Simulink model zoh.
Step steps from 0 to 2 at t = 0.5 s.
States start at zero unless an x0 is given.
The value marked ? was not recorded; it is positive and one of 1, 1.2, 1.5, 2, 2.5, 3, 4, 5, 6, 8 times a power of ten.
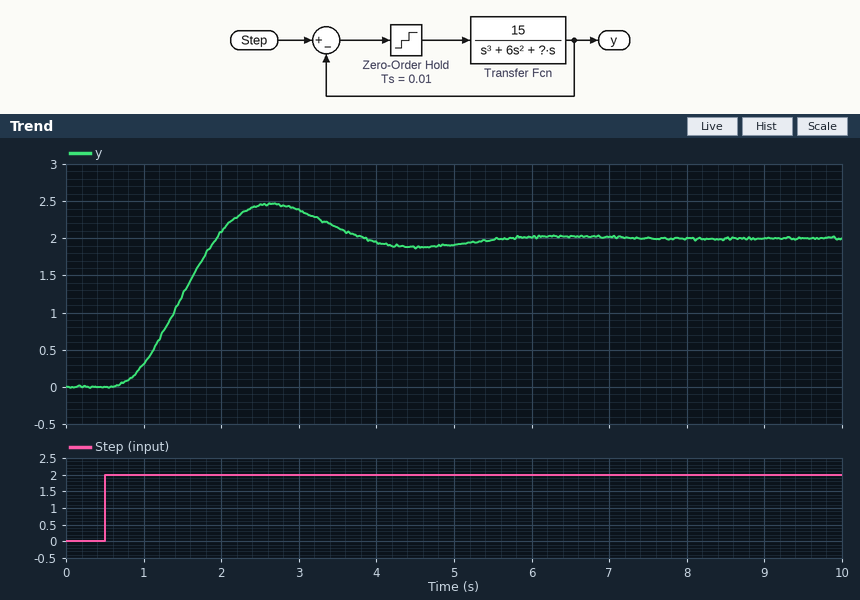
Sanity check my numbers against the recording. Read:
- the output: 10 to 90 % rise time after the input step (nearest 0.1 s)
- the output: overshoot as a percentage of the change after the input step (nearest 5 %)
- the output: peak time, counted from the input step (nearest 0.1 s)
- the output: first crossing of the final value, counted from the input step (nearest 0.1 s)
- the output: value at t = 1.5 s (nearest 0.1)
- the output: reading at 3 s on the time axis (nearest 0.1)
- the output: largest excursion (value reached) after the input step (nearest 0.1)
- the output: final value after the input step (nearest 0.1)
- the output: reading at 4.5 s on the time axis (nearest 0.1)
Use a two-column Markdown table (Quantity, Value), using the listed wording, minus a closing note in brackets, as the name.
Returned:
| Quantity | Value |
|---|---|
| the output: 10 to 90 % rise time after the input step | 0.9 s |
| the output: overshoot as a percentage of the change after the input step | 25 % |
| the output: peak time, counted from the input step | 2.1 s |
| the output: first crossing of the final value, counted from the input step | 1.4 s |
| the output: value at t = 1.5 s | 1.2 |
| the output: reading at 3 s on the time axis | 2.4 |
| the output: largest excursion (value reached) after the input step | 2.5 |
| the output: final value after the input step | 2.0 |
| the output: reading at 4.5 s on the time axis | 1.9 |
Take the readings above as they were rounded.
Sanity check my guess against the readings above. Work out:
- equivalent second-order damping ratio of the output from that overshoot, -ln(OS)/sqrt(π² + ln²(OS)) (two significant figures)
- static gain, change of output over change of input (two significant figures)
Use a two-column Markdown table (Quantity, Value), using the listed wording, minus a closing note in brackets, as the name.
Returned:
| Quantity | Value |
|---|---|
| equivalent second-order damping ratio of the output from that overshoot, -ln(OS)/sqrt(π² + ln²(OS)) | 0.40 |
| static gain, change of output over change of input | 1.0 |
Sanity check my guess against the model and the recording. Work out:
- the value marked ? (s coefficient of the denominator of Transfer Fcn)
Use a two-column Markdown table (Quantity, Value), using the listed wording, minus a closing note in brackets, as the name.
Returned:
| Quantity | Value |
|---|---|
| the value marked ? | 10 |
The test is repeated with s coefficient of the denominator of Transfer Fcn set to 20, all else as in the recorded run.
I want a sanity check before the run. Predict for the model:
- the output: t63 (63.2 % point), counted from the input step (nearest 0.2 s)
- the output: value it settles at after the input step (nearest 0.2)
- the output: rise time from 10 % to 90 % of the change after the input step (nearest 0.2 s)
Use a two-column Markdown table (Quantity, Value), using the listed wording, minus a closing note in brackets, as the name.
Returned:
| Quantity | Value |
|---|---|
| the output: t63 (63.2 % point), counted from the input step | 1.4 s |
| the output: value it settles at after the input step | 2.0 |
| the output: rise time from 10 % to 90 % of the change after the input step | 2.2 s |
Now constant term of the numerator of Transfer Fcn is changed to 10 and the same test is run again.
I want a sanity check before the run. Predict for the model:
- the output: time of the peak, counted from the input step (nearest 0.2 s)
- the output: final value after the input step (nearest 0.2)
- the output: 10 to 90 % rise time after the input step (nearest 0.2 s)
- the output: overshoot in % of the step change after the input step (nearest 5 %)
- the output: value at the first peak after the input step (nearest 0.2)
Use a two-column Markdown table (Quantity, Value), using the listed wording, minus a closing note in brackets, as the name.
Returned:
| Quantity | Value |
|---|---|
| the output: time of the peak, counted from the input step | 2.8 s |
| the output: final value after the input step | 2.0 |
| the output: 10 to 90 % rise time after the input step | 1.2 s |
| the output: overshoot in % of the step change after the input step | 10 % |
| the output: value at the first peak after the input step | 2.2 |
